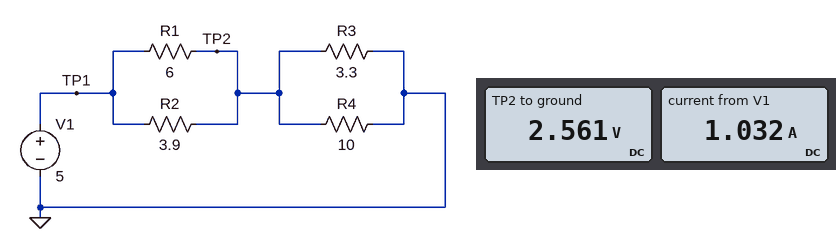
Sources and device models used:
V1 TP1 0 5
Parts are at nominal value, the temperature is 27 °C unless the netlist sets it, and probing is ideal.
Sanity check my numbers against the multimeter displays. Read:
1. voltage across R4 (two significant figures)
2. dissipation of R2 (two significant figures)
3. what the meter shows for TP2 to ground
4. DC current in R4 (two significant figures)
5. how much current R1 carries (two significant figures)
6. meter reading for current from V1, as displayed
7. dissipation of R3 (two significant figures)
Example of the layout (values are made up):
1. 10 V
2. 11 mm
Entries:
1. 2.6 V
2. 1.5 W
3. 2.561 V
4. 260 mA
5. 410 mA
6. 1.032 A
7. 2.0 W
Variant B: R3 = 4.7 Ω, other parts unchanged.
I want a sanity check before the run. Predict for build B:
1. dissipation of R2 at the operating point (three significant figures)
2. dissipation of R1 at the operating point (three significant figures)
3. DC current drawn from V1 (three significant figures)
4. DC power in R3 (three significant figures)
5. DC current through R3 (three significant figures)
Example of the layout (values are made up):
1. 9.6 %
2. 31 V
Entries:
1. 1.16 W
2. 753 mW
3. 899 mA
4. 1.76 W
5. 612 mA
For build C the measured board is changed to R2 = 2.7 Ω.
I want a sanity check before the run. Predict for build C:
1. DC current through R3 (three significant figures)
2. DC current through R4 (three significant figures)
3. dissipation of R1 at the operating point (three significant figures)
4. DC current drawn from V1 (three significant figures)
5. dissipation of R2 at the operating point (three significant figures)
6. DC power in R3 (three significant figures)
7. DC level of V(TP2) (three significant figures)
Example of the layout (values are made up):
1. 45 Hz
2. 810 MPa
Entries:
1. 866 mA
2. 286 mA
3. 766 mW
4. 1.15 A
5. 1.70 W
6. 2.47 W
7. 2.86 V
